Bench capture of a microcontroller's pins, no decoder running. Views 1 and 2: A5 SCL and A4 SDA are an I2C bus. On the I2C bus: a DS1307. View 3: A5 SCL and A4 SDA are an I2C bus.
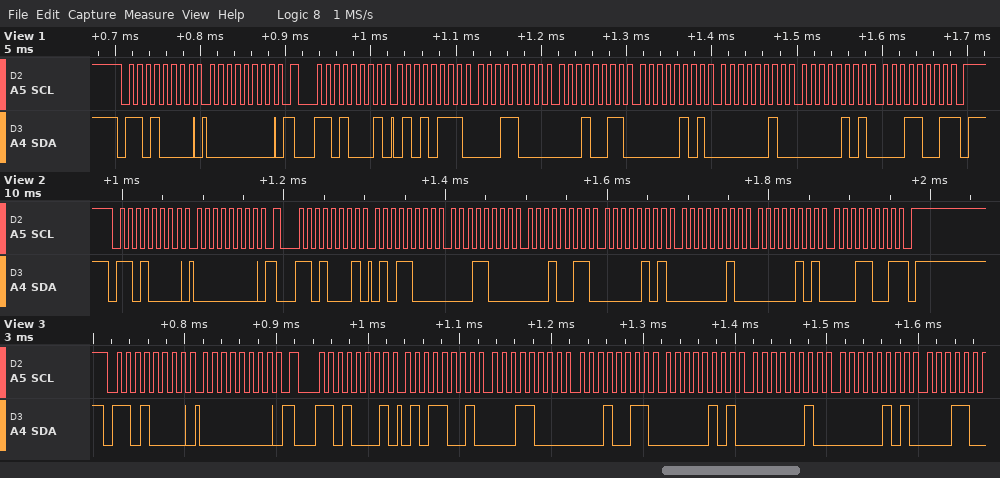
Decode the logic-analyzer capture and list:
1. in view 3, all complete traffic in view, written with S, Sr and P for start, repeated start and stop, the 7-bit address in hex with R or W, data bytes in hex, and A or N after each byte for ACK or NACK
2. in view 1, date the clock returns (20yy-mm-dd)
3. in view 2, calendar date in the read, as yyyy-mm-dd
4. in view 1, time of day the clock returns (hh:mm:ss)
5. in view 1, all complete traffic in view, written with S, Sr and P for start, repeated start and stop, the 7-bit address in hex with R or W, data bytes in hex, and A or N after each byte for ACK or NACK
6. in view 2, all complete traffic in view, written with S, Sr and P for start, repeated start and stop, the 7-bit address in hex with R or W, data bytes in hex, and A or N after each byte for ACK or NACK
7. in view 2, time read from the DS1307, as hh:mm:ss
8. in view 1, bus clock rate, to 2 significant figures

S 68W A 00 A Sr 68R A 59 A 18 A 13 A 05 A 02 A 05 A
2019-05-02
2019-05-02
13:18:57
S 68W A 00 A Sr 68R A 57 A 18 A 13 A 05 A 02 A 05 A 19 N P
S 68W A 00 A Sr 68R A 58 A 18 A 13 A 05 A 02 A 05 A 19 N P
13:18:58
100 kHz
